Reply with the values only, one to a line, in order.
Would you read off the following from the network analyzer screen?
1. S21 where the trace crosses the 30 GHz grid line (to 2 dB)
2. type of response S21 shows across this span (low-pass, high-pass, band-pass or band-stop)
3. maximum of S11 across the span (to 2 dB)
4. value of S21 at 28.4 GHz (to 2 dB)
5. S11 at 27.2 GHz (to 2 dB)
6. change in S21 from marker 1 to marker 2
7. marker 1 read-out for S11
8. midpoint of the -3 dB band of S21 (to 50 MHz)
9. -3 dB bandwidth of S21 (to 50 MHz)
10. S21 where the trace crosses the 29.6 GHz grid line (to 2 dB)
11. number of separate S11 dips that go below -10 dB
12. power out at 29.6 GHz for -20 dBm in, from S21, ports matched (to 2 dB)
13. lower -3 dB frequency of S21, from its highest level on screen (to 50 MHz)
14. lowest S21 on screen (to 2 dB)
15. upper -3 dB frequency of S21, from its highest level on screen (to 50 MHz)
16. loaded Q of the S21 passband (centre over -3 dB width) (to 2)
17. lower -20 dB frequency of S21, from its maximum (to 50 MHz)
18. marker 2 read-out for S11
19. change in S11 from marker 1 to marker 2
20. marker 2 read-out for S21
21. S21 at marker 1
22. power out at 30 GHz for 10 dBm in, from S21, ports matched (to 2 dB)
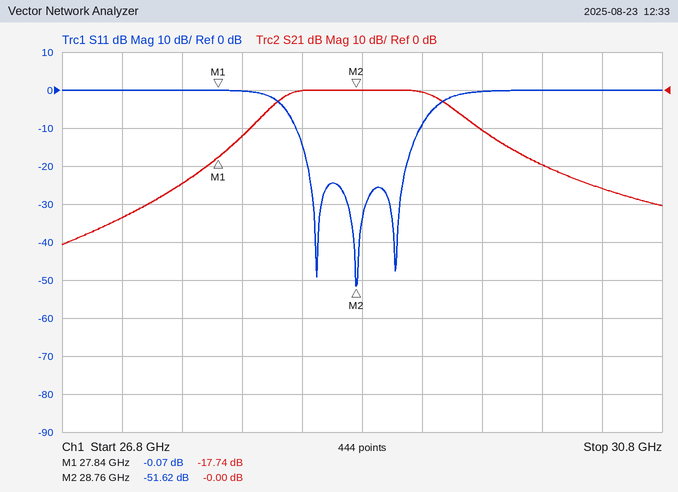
-20 dB
band-pass
0 dB
0 dB
0 dB
17.74 dB
-0.07 dB
28.80 GHz
1.10 GHz
-10 dB
3
-30 dBm
28.25 GHz
-40 dB
29.35 GHz
26
27.75 GHz
-51.62 dB
-51.55 dB
-0.00 dB
-17.74 dB
-10 dBm
